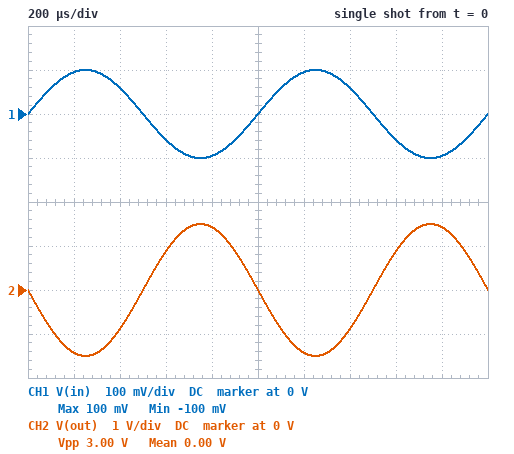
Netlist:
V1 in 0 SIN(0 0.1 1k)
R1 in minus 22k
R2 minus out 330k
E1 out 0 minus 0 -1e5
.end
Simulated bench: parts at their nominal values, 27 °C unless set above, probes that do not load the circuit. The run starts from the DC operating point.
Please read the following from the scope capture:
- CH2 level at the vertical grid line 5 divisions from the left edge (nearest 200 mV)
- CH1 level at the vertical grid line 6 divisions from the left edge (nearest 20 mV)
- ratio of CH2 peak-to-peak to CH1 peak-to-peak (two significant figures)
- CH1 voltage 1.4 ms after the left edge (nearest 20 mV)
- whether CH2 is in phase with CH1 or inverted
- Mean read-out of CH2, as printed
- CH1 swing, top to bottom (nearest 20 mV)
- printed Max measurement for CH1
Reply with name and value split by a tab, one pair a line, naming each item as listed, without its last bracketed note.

CH2 level at the vertical grid line 5 divisions from the left edge	0 V
CH1 level at the vertical grid line 6 divisions from the left edge	100 mV
ratio of CH2 peak-to-peak to CH1 peak-to-peak	15
CH1 voltage 1.4 ms after the left edge	60 mV
whether CH2 is in phase with CH1 or inverted	inverted
Mean read-out of CH2, as printed	0.00 V
CH1 swing, top to bottom	200 mV
printed Max measurement for CH1	100 mV
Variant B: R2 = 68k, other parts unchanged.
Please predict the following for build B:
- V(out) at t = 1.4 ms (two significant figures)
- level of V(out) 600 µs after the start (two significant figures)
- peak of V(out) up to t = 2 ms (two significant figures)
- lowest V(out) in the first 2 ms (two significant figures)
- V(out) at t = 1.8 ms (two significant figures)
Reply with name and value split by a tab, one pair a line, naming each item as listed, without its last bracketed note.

V(out) at t = 1.4 ms	-180 mV
level of V(out) 600 µs after the start	180 mV
peak of V(out) up to t = 2 ms	310 mV
lowest V(out) in the first 2 ms	-310 mV
V(out) at t = 1.8 ms	290 mV
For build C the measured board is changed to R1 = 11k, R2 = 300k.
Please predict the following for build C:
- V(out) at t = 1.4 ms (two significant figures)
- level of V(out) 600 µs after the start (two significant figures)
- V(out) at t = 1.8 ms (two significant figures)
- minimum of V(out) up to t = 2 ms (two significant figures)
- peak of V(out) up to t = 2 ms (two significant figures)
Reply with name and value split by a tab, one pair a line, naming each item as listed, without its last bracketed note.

V(out) at t = 1.4 ms	-1.6 V
level of V(out) 600 µs after the start	1.6 V
V(out) at t = 1.8 ms	2.6 V
minimum of V(out) up to t = 2 ms	-2.7 V
peak of V(out) up to t = 2 ms	2.7 V
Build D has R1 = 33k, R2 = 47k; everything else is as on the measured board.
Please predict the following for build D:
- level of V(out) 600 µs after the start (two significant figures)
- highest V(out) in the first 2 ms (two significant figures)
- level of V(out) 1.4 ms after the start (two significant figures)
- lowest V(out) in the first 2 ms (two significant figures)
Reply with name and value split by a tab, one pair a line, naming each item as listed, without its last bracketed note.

level of V(out) 600 µs after the start	84 mV
highest V(out) in the first 2 ms	140 mV
level of V(out) 1.4 ms after the start	-84 mV
lowest V(out) in the first 2 ms	-140 mV
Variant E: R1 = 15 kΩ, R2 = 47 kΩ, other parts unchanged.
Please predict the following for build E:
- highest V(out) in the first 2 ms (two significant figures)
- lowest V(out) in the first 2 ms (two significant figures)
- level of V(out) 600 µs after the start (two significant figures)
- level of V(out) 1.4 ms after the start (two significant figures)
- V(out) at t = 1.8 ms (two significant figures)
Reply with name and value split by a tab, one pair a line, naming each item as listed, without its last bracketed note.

highest V(out) in the first 2 ms	310 mV
lowest V(out) in the first 2 ms	-310 mV
level of V(out) 600 µs after the start	180 mV
level of V(out) 1.4 ms after the start	-180 mV
V(out) at t = 1.8 ms	300 mV
